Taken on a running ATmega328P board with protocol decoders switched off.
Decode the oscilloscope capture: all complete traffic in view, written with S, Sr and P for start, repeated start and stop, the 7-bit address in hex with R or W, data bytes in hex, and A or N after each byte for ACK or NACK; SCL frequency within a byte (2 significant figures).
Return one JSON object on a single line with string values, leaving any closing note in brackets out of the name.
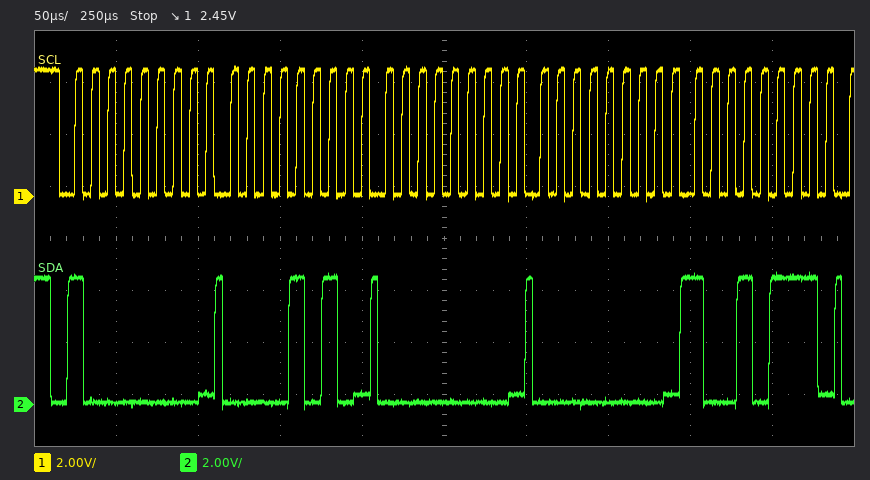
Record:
{"all complete traffic in view, written with S, Sr and P for start, repeated start and stop, the 7-bit address in hex with R or W, data bytes in hex, and A or N after each byte for ACK or NACK": "S 40W A 0A A 00 A 00 A 97 A", "SCL frequency within a byte": "100 kHz"}
